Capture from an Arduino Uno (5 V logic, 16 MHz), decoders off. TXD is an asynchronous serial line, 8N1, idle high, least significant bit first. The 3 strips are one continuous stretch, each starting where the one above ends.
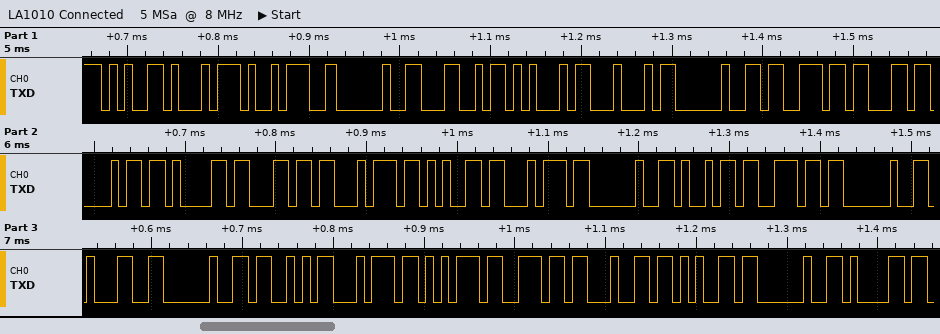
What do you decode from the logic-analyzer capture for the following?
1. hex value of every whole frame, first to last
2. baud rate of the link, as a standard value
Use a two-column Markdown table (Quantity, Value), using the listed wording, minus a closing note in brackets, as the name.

| Quantity | Value |
|---|---|
| hex value of every whole frame, first to last | 65 74 3A 20 4C 45 44 20 73 63 68 61 6C 74 65 74 20 69 6E 20 31 20 53 74 75 6E 64 65 20 61 |
| baud rate of the link, as a standard value | 115200 baud |
